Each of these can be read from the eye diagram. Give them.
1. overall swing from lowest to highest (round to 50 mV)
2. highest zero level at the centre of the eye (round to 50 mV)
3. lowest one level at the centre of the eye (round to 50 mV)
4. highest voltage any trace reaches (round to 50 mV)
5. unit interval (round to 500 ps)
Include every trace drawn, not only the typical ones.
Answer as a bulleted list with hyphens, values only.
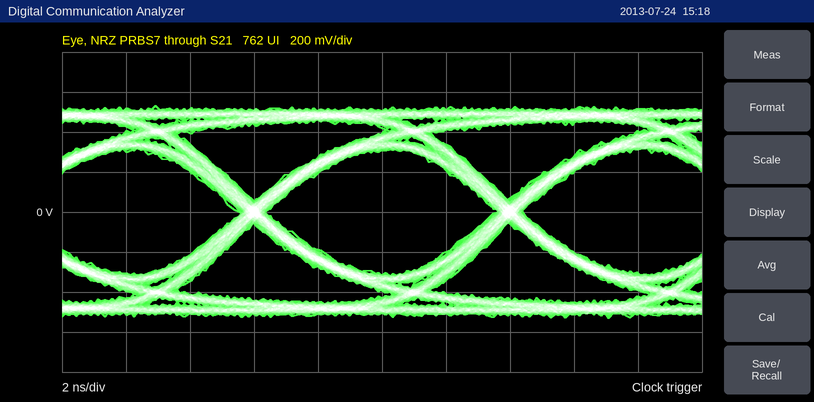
- 1.05 V
- -300 mV
- 300 mV
- 550 mV
- 8.0 ns
